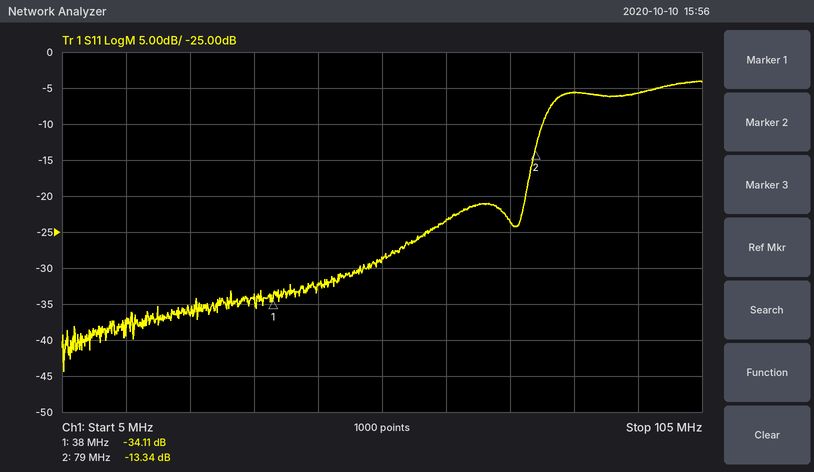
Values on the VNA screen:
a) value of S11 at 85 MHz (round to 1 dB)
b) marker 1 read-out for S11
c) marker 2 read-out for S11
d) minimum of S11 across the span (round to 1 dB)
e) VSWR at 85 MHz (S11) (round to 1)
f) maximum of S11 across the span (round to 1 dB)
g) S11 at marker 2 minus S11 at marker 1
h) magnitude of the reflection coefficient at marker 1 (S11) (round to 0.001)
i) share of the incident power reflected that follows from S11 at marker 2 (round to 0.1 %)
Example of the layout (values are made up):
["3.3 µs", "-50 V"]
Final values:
["-6 dB", "-34.11 dB", "-13.34 dB", "-44 dB", "3", "-4 dB", "20.77 dB", "0.020", "4.6 %"]
